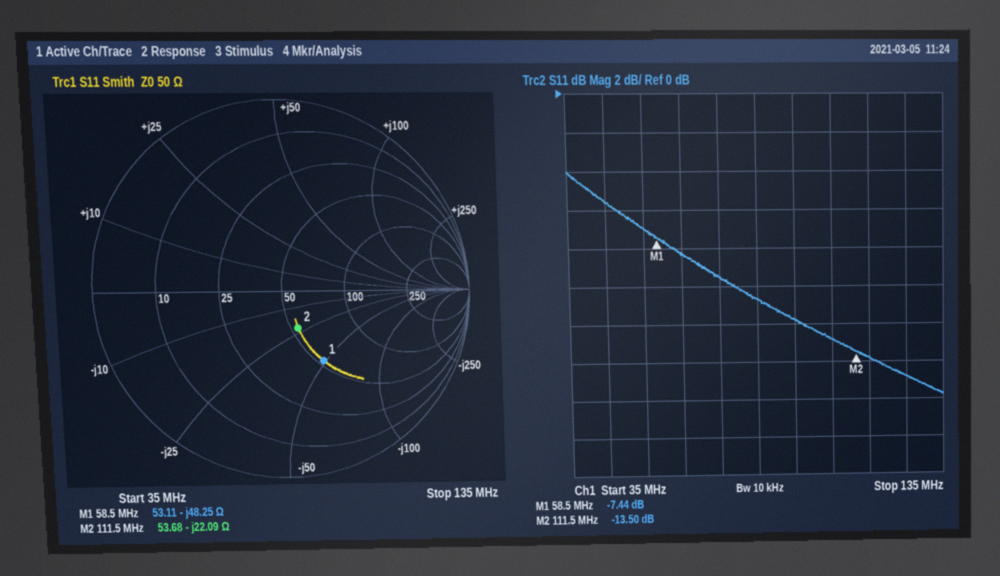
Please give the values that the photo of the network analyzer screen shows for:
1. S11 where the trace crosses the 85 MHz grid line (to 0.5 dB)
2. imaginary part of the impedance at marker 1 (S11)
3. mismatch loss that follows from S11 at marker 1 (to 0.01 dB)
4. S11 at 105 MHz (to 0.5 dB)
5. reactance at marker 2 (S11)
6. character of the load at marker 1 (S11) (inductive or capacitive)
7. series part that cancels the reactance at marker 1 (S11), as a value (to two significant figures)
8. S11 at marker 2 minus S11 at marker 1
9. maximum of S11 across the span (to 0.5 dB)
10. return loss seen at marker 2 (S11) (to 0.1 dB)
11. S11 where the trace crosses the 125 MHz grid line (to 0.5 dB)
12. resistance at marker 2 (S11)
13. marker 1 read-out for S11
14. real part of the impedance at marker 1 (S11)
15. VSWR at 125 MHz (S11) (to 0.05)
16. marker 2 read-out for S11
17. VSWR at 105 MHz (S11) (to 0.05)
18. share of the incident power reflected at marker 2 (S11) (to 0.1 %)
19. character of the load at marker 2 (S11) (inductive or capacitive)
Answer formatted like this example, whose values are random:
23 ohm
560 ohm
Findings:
-10.5 dB
-48.25 Ω
0.86 dB
-13.0 dB
-22.09 Ω
capacitive
130 nH
-6.06 dB
-4.0 dB
13.5 dB
-15.0 dB
53.68 Ω
-7.44 dB
53.11 Ω
1.45
-13.50 dB
1.60
4.5 %
capacitive
